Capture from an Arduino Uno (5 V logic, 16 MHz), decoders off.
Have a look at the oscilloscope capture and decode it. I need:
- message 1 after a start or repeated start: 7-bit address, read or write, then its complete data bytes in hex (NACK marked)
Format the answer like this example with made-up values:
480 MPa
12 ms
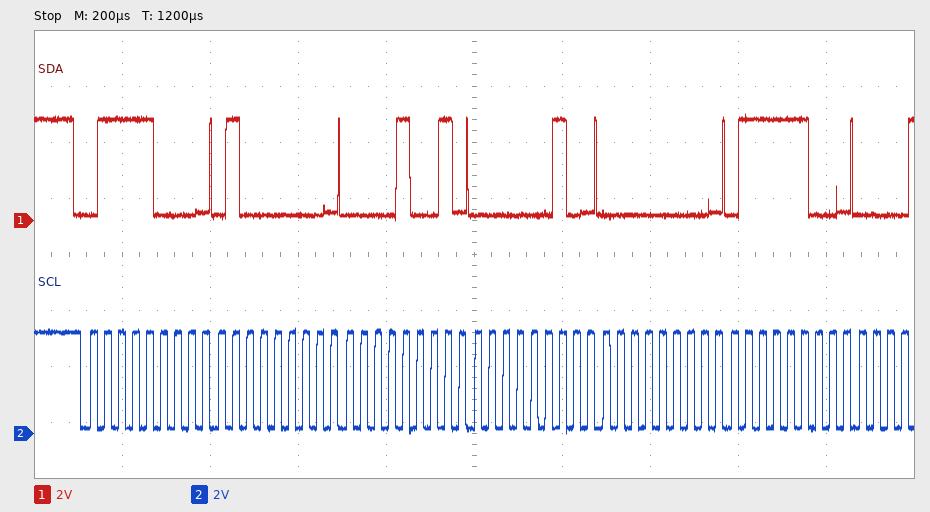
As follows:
0x3C write: 40 09 02 00 7C
